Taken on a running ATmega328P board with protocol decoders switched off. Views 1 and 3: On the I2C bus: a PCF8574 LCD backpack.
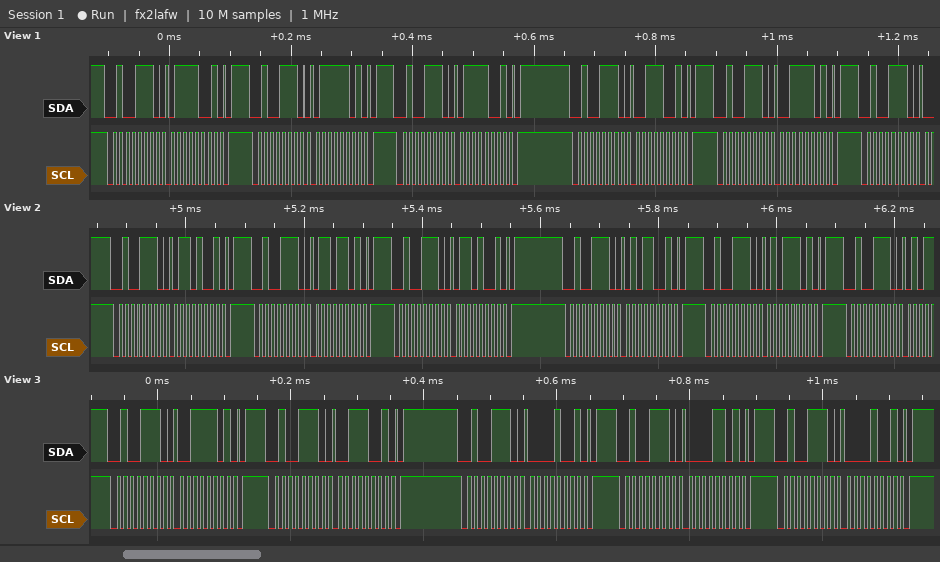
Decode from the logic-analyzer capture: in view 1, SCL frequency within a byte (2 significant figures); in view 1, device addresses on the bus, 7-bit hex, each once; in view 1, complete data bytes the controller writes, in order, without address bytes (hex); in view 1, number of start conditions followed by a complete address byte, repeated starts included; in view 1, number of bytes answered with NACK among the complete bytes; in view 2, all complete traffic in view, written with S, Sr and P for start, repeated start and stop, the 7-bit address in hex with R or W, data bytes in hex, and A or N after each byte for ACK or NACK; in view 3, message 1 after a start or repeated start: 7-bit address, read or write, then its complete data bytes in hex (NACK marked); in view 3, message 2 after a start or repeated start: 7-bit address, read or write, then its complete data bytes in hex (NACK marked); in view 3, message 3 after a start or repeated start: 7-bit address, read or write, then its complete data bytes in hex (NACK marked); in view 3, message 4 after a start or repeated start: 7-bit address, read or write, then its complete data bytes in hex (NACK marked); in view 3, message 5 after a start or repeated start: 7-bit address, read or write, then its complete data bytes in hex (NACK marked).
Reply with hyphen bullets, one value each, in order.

- 100 kHz
- 0x27
- 79 7D 79 39 3D
- 6
- 0
- S 27W A 69 A P S 27W A 6D A P S 27W A 69 A P S 27W A 59 A P S 27W A 5D A P S 27W A
- 0x27 write: 3D
- 0x27 write: 39
- 0x27 write: 09
- 0x27 write: 0D
- 0x27 write: 09
